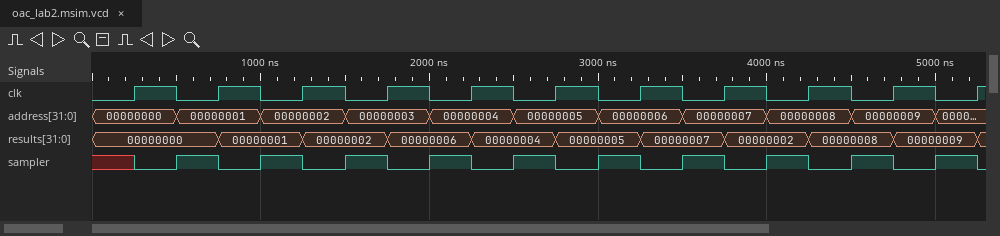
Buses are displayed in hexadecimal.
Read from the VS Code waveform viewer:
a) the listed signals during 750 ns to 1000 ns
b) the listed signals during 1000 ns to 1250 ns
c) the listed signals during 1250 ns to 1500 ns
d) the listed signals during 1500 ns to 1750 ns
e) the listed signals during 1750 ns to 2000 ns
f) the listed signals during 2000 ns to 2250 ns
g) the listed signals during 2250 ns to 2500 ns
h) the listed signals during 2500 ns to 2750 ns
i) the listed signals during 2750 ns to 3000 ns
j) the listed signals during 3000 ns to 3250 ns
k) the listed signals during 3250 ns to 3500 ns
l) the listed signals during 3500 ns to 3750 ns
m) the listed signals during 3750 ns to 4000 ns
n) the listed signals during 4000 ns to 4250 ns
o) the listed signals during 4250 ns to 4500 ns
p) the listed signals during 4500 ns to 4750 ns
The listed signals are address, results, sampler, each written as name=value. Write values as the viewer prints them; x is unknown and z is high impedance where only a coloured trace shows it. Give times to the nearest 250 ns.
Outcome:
address=00000001, results=00000001, sampler=0
address=00000002, results=00000001, sampler=1
address=00000002, results=00000002, sampler=0
address=00000003, results=00000002, sampler=1
address=00000003, results=00000006, sampler=0
address=00000004, results=00000006, sampler=1
address=00000004, results=00000004, sampler=0
address=00000005, results=00000004, sampler=1
address=00000005, results=00000005, sampler=0
address=00000006, results=00000005, sampler=1
address=00000006, results=00000007, sampler=0
address=00000007, results=00000007, sampler=1
address=00000007, results=00000002, sampler=0
address=00000008, results=00000002, sampler=1
address=00000008, results=00000008, sampler=0
address=00000009, results=00000008, sampler=1
